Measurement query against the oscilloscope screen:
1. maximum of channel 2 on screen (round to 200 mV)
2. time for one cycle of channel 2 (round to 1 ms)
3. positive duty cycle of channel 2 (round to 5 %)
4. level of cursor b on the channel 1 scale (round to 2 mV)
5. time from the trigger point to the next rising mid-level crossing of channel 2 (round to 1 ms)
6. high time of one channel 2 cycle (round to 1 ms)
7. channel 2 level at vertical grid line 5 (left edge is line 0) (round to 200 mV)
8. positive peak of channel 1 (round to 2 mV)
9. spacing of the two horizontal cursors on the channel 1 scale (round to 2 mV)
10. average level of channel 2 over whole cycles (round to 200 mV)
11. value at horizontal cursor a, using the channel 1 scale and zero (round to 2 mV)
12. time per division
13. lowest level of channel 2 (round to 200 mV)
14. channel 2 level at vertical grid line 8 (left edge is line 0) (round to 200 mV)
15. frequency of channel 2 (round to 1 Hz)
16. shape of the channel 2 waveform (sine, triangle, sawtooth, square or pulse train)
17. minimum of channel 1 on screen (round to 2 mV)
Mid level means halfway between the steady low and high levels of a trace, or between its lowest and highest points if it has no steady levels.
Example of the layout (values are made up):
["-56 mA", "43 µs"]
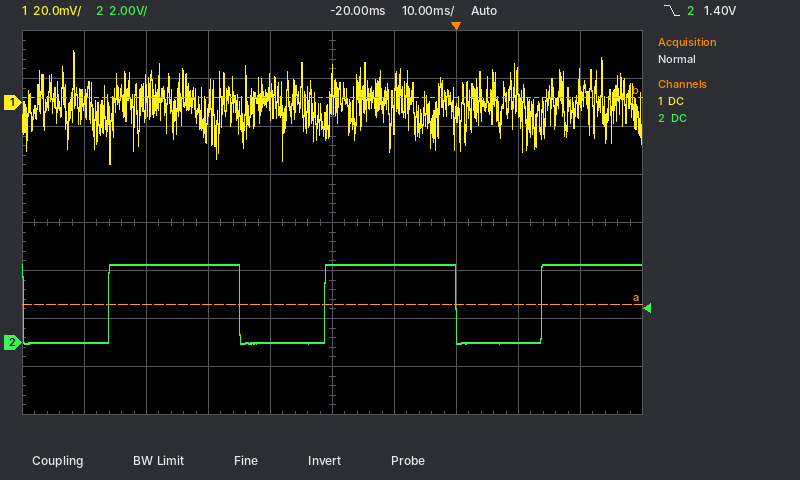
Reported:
["3.2 V", "35 ms", "60 %", "2 mV", "14 ms", "21 ms", "3.2 V", "22 mV", "86 mV", "2.0 V", "-84 mV", "10 ms", "0.0 V", "0.0 V", "29 Hz", "pulse train", "-26 mV"]
